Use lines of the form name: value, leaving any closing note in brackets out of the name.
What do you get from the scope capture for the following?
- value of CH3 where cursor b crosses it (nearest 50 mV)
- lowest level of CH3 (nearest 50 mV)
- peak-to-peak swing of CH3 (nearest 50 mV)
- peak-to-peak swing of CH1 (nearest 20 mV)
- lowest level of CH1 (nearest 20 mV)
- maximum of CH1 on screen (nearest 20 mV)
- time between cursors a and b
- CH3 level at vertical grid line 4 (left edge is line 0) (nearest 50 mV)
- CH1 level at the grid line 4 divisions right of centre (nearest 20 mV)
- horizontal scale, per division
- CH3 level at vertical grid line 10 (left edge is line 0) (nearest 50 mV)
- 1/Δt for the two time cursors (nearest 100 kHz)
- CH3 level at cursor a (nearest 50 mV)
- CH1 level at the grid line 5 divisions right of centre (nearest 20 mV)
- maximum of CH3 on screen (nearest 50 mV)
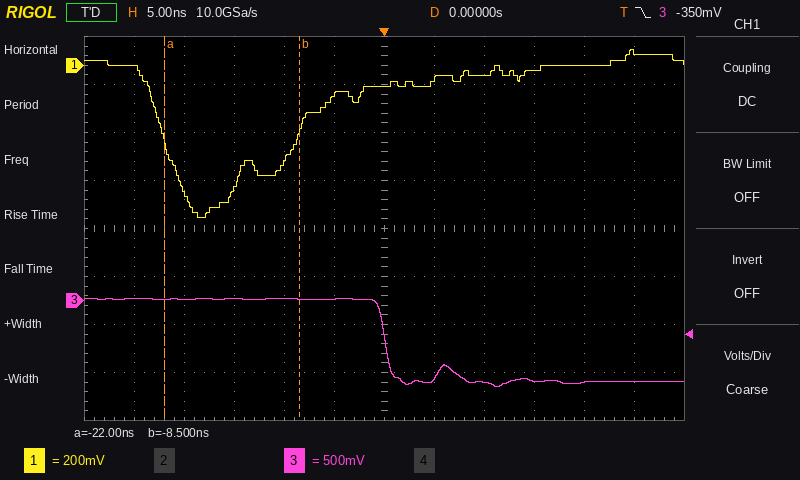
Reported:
value of CH3 where cursor b crosses it: 0 mV
lowest level of CH3: -900 mV
peak-to-peak swing of CH3: 900 mV
peak-to-peak swing of CH1: 700 mV
lowest level of CH1: -640 mV
maximum of CH1 on screen: 60 mV
time between cursors a and b: 13.5 ns
CH3 level at vertical grid line 4 (left edge is line 0): 0 mV
CH1 level at the grid line 4 divisions right of centre: 0 mV
horizontal scale, per division: 5 ns
CH3 level at vertical grid line 10 (left edge is line 0): -850 mV
1/Δt for the two time cursors: 74.1 MHz
CH3 level at cursor a: 0 mV
CH1 level at the grid line 5 divisions right of centre: 60 mV
maximum of CH3 on screen: 0 mV
